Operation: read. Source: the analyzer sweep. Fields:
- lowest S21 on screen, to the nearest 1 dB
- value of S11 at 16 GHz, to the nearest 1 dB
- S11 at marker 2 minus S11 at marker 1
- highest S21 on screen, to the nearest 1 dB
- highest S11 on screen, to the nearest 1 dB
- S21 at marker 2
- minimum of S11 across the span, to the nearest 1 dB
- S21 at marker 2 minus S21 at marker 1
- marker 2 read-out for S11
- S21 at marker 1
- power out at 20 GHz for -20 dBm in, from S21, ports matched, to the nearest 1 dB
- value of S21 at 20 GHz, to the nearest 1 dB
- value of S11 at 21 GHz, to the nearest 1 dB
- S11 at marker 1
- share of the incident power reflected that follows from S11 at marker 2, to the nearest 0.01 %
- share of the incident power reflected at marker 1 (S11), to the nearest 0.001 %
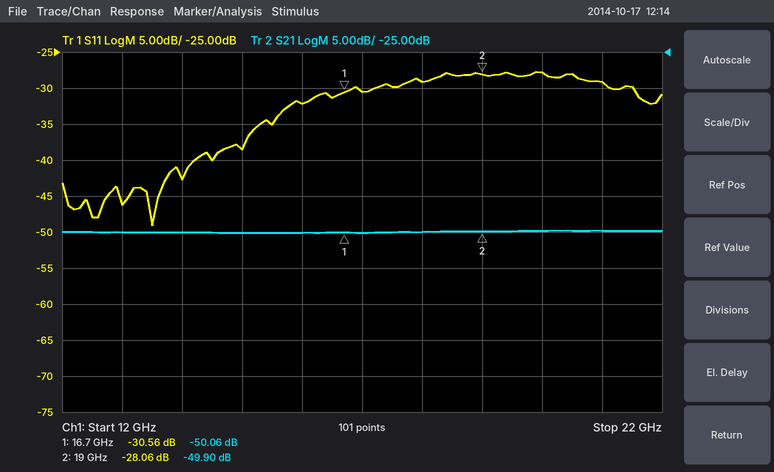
-50 dB
-32 dB
2.50 dB
-50 dB
-28 dB
-49.90 dB
-49 dB
0.16 dB
-28.06 dB
-50.06 dB
-70 dBm
-50 dB
-29 dB
-30.56 dB
0.16 %
0.088 %
